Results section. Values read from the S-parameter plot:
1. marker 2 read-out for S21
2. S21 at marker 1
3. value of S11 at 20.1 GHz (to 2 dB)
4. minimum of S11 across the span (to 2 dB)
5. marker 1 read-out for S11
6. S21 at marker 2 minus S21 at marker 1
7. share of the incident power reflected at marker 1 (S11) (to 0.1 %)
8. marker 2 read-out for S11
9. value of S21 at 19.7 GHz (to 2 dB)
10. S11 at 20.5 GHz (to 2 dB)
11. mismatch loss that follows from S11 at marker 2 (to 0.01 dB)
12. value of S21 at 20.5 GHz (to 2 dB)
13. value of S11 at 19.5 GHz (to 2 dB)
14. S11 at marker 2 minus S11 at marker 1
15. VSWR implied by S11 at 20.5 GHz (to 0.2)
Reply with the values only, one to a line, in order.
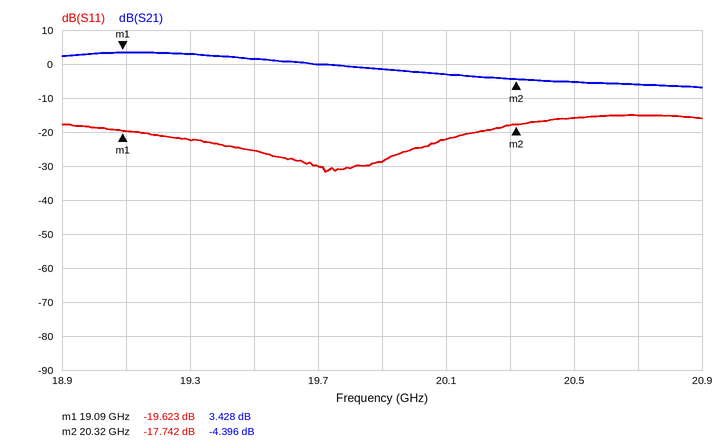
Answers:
-4.396 dB
3.428 dB
-22 dB
-32 dB
-19.623 dB
-7.824 dB
1.1 %
-17.742 dB
0 dB
-16 dB
0.07 dB
-6 dB
-26 dB
1.881 dB
1.4
